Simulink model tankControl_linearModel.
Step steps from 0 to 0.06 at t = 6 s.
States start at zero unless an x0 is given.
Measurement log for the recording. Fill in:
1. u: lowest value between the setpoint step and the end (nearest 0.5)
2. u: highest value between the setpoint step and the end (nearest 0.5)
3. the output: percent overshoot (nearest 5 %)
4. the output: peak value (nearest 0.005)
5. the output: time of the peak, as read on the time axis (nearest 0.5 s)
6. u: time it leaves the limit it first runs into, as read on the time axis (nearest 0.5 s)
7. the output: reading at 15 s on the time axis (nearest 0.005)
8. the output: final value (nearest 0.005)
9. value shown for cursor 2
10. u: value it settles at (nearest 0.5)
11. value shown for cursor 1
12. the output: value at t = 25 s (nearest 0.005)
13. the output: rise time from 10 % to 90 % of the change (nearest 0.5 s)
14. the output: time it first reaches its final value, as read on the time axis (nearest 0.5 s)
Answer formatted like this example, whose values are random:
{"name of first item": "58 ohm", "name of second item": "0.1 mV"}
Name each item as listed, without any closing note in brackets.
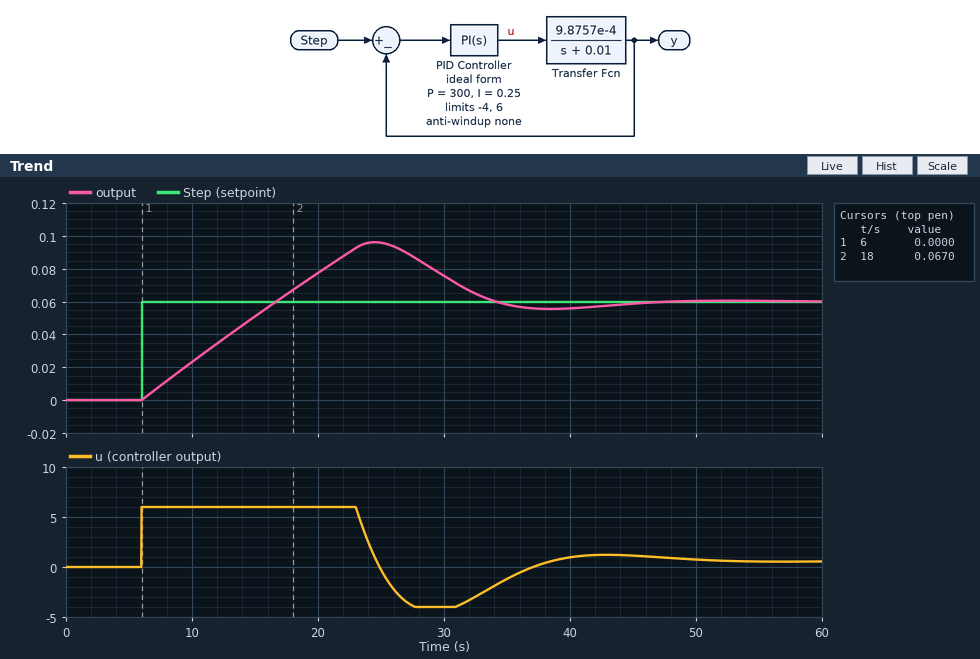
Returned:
{"u: lowest value between the setpoint step and the end": "-4.0", "u: highest value between the setpoint step and the end": "6.0", "the output: percent overshoot": "60 %", "the output: peak value": "0.095", "the output: time of the peak, as read on the time axis": "24.5 s", "u: time it leaves the limit it first runs into, as read on the time axis": "23.0 s", "the output: reading at 15 s on the time axis": "0.050", "the output: final value": "0.060", "value shown for cursor 2": "0.0670", "u: value it settles at": "0.5", "value shown for cursor 1": "0.0000", "the output: value at t = 25 s": "0.095", "the output: rise time from 10 % to 90 % of the change": "8.5 s", "the output: time it first reaches its final value, as read on the time axis": "16.5 s"}
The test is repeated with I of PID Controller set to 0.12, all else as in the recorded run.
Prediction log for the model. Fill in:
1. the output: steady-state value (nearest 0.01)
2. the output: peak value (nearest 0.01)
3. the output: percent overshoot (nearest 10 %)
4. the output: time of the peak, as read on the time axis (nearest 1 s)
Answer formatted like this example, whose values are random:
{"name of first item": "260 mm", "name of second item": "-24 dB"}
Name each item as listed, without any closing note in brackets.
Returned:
{"the output: steady-state value": "0.06", "the output: peak value": "0.08", "the output: percent overshoot": "40 %", "the output: time of the peak, as read on the time axis": "23 s"}
